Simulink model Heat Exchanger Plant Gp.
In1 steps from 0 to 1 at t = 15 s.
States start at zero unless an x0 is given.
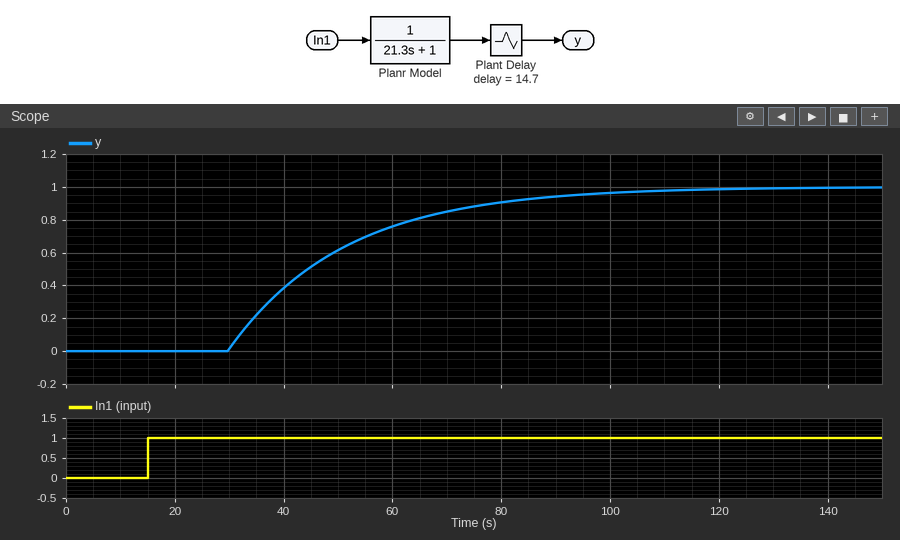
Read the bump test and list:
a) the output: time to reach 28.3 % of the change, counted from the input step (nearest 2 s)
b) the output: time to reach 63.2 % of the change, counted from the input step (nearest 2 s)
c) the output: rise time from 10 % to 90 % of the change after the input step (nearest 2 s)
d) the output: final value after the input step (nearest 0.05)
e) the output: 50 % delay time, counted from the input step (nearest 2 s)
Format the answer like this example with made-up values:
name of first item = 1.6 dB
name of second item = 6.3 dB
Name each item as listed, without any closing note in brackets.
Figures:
the output: time to reach 28.3 % of the change, counted from the input step = 22 s
the output: time to reach 63.2 % of the change, counted from the input step = 36 s
the output: rise time from 10 % to 90 % of the change after the input step = 46 s
the output: final value after the input step = 1.00
the output: 50 % delay time, counted from the input step = 30 s
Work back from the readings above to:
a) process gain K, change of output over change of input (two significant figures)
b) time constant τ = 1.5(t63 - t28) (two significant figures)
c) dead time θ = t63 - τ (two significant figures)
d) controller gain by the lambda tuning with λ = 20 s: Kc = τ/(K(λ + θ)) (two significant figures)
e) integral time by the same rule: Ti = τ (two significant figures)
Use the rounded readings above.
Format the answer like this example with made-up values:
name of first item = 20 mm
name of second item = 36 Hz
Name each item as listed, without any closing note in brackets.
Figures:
process gain K, change of output over change of input = 1.0
time constant τ = 1.5(t63 - t28) = 21 s
dead time θ = t63 - τ = 15 s
controller gain by the lambda tuning with λ = 20 s: Kc = τ/(K(λ + θ)) = 0.60
integral time by the same rule: Ti = τ = 21 s
